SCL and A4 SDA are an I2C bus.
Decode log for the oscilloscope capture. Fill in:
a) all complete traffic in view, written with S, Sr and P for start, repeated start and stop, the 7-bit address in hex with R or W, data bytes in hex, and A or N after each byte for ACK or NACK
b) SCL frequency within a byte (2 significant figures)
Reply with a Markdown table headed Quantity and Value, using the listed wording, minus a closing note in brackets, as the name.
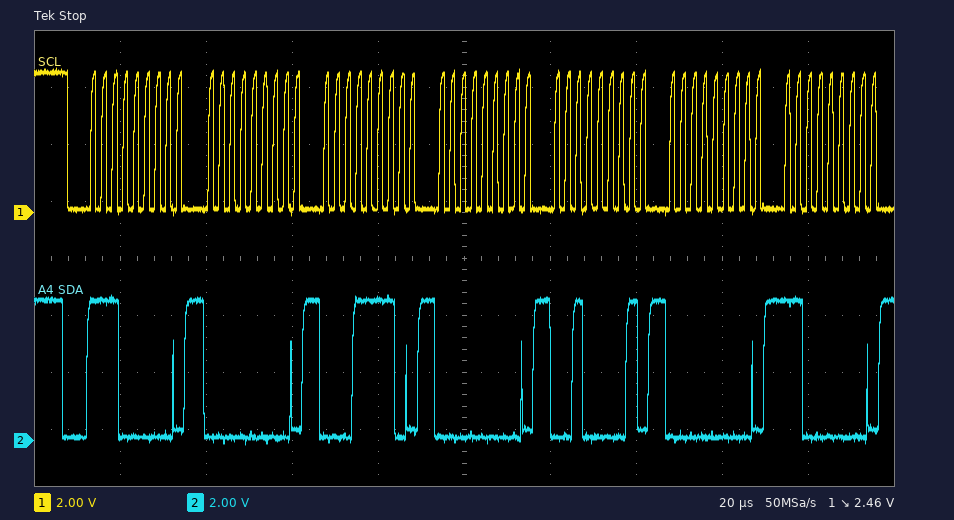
| Quantity | Value |
|---|---|
| all complete traffic in view, written with S, Sr and P for start, repeated start and stop, the 7-bit address in hex with R or W, data bytes in hex, and A or N after each byte for ACK or NACK | S 70W A 00 A 1E A 00 A 21 A 00 A C0 A |
| SCL frequency within a byte | 400 kHz |
